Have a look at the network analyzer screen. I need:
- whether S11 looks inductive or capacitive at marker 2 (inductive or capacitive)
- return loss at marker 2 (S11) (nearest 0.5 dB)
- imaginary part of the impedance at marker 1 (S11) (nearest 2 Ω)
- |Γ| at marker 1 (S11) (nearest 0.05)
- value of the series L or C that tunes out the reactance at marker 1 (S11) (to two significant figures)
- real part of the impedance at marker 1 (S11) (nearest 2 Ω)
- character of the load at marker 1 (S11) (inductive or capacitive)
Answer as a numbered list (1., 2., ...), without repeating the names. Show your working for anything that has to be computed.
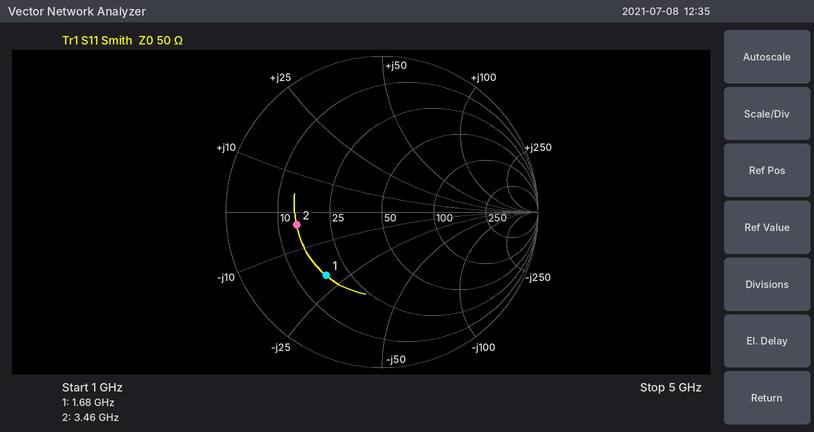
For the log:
1. capacitive
2. 5.0 dB
3. -20 Ω
4. 0.55
5. L = 20 Ω/(2π × 1.68 GHz) ≈ 1.9 nH
6. 18 Ω
7. capacitive
